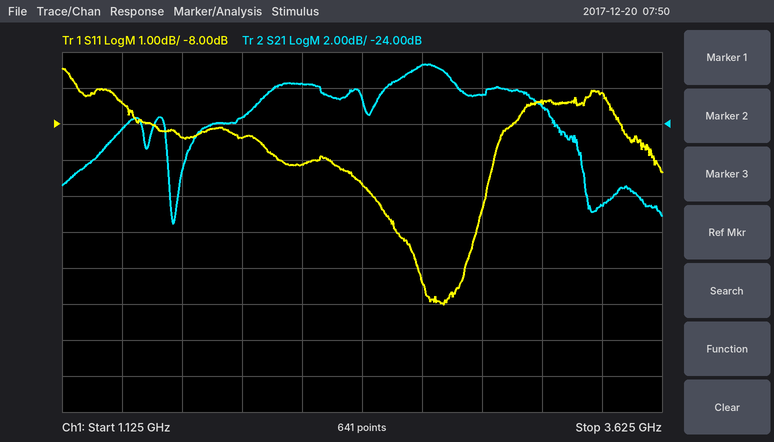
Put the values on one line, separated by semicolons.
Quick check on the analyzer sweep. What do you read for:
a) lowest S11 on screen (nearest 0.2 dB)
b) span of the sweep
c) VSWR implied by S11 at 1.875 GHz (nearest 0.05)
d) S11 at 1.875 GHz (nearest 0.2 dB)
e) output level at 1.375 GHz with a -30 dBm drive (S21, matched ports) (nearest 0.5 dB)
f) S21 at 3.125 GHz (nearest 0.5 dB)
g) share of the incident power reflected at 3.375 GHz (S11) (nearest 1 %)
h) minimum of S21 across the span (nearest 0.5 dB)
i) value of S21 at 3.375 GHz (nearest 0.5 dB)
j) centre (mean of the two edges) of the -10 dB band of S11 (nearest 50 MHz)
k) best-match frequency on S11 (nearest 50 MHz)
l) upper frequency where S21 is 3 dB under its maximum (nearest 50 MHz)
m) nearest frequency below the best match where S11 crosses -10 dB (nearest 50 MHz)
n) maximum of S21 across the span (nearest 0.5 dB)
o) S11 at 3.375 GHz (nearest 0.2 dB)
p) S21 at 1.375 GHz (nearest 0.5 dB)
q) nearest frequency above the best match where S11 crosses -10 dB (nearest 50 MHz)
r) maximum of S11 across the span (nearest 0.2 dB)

-13.0 dB; 2.5 GHz; 2.25; -8.4 dB; -54.5 dBm; -23.0 dB; 19 %; -29.5 dB; -28.5 dB; 2.65 GHz; 2.70 GHz; 3.15 GHz; 2.40 GHz; -20.5 dB; -7.2 dB; -24.5 dB; 2.90 GHz; -6.4 dB
